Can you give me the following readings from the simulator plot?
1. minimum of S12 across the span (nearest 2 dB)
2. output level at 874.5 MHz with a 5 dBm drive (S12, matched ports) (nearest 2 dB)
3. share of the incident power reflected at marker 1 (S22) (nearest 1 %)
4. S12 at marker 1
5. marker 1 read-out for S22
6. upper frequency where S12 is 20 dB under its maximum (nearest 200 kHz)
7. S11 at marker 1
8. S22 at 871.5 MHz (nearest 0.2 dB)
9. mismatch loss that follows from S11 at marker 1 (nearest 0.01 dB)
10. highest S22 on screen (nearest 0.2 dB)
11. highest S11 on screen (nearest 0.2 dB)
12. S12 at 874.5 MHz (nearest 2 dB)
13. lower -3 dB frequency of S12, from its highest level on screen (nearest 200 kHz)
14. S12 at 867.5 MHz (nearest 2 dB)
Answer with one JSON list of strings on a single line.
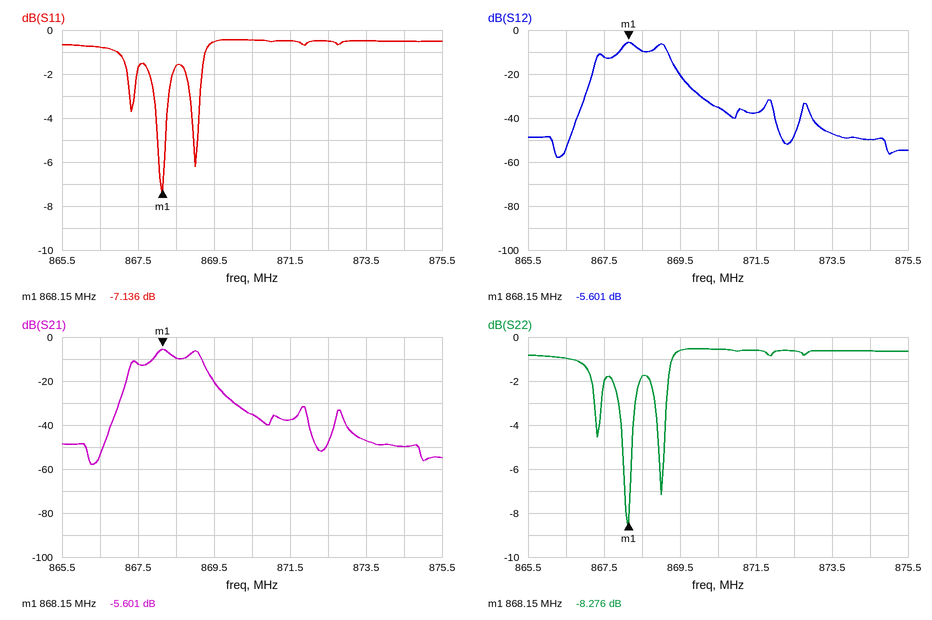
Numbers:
["-58 dB", "-44 dBm", "15 %", "-5.601 dB", "-8.276 dB", "869.8 MHz", "-7.136 dB", "-0.6 dB", "0.93 dB", "-0.6 dB", "-0.4 dB", "-50 dB", "868.0 MHz", "-12 dB"]
